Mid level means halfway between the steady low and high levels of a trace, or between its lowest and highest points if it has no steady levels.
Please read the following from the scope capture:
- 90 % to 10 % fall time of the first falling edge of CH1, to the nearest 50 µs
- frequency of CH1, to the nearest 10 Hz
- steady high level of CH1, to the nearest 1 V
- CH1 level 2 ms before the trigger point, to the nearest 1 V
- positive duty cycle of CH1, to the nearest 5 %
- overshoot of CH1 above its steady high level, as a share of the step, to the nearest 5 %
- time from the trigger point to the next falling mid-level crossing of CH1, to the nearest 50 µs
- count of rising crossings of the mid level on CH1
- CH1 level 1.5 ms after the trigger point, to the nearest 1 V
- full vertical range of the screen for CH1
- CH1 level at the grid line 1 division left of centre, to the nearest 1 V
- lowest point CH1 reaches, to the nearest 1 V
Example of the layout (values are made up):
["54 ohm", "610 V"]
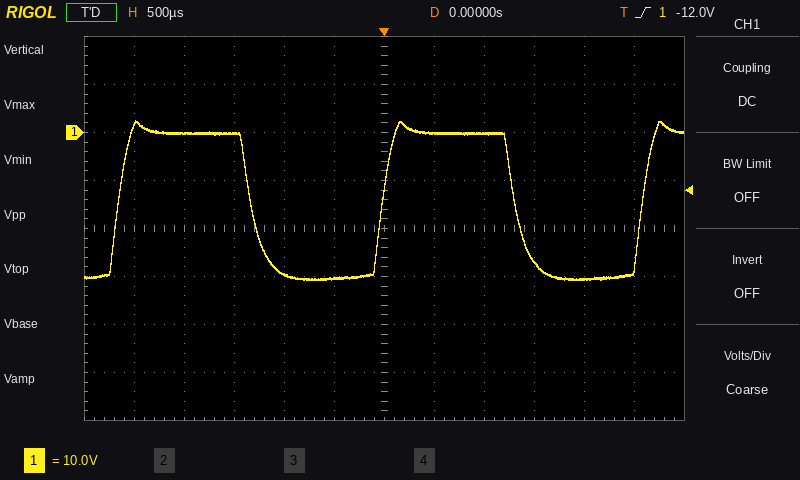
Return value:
["300 µs", "380 Hz", "0 V", "0 V", "50 %", "10 %", "1.30 ms", "3", "-27 V", "80 V", "-30 V", "-31 V"]
